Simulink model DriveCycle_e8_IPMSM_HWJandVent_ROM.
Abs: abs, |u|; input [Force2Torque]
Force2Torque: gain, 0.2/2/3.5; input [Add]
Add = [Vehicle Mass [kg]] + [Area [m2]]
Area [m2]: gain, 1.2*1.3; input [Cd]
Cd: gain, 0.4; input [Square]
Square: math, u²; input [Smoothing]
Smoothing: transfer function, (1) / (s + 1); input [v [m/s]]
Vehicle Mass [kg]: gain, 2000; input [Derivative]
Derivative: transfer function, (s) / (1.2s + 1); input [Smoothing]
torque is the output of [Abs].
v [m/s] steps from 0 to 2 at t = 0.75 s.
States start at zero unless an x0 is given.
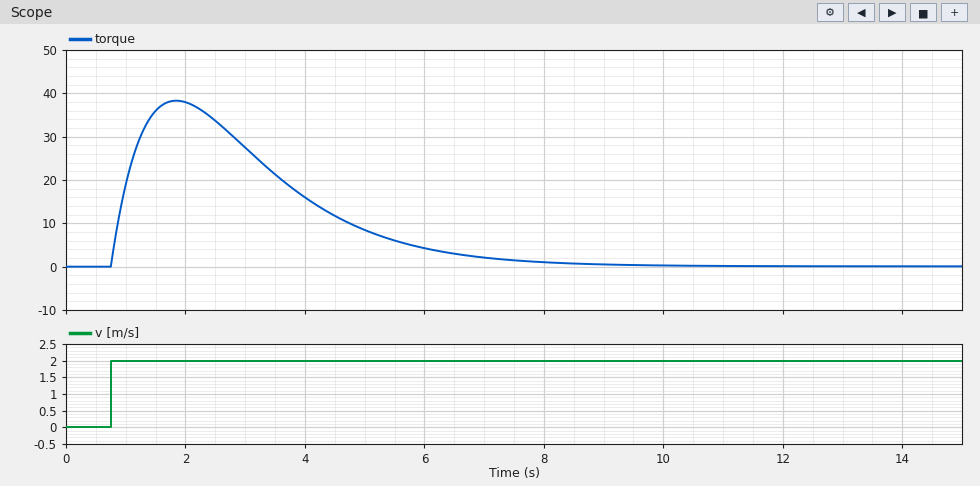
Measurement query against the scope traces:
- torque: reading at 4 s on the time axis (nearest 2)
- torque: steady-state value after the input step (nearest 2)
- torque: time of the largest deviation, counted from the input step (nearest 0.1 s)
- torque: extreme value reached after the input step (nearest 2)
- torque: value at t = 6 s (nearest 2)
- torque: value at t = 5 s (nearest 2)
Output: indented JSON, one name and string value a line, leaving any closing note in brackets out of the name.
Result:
{
  "torque: reading at 4 s on the time axis": "16",
  "torque: steady-state value after the input step": "0",
  "torque: time of the largest deviation, counted from the input step": "1.1 s",
  "torque: extreme value reached after the input step": "38",
  "torque: value at t = 6 s": "4",
  "torque: value at t = 5 s": "8"
}
